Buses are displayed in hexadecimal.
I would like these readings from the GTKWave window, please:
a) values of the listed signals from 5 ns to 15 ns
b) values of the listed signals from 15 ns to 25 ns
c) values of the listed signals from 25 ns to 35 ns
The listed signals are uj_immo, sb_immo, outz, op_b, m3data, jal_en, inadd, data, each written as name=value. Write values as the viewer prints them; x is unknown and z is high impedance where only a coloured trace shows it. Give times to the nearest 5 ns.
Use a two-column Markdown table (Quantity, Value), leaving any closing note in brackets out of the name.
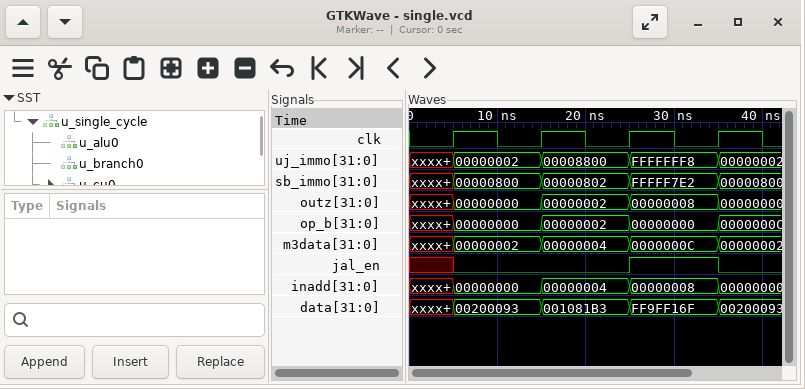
| Quantity | Value |
|---|---|
| values of the listed signals from 5 ns to 15 ns | uj_immo=00000002, sb_immo=00000800, outz=00000000, op_b=00000000, m3data=00000002, jal_en=0, inadd=00000000, data=00200093 |
| values of the listed signals from 15 ns to 25 ns | uj_immo=00008800, sb_immo=00000802, outz=00000002, op_b=00000002, m3data=00000004, jal_en=0, inadd=00000004, data=001081B3 |
| values of the listed signals from 25 ns to 35 ns | uj_immo=FFFFFFF8, sb_immo=FFFFF7E2, outz=00000008, op_b=00000000, m3data=0000000C, jal_en=1, inadd=00000008, data=FF9FF16F |
